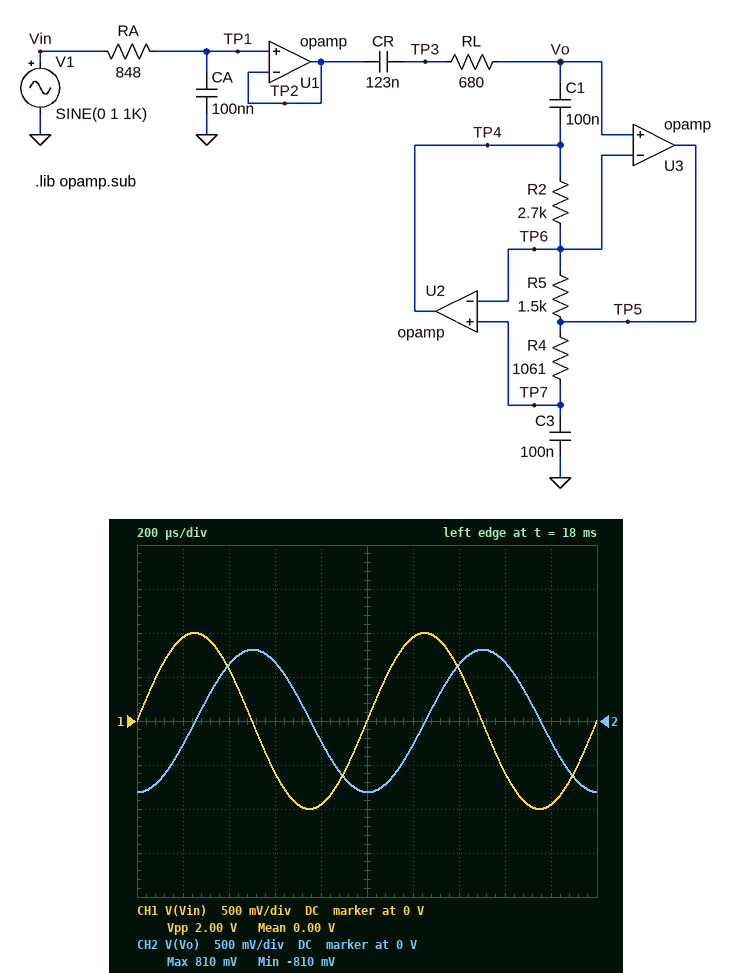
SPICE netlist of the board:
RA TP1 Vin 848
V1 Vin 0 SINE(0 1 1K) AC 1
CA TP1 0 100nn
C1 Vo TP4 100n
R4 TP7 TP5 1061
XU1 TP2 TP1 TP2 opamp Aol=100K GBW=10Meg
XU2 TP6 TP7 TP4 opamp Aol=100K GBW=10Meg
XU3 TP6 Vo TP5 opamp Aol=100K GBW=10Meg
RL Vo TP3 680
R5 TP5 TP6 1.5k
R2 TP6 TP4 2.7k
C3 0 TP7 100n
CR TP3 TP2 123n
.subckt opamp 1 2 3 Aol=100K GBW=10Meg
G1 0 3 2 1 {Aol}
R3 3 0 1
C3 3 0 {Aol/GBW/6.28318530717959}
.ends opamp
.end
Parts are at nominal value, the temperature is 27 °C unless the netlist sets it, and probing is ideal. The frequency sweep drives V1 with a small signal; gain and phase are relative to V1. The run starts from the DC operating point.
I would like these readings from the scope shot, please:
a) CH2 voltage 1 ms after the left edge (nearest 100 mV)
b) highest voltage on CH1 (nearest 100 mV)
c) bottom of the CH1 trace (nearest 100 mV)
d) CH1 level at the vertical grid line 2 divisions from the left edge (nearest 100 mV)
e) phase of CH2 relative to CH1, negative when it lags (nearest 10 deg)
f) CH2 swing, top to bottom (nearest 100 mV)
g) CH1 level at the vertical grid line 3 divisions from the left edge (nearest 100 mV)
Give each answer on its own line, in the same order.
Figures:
-800 mV
1.0 V
-1.0 V
600 mV
-90 deg
1.6 V
-600 mV
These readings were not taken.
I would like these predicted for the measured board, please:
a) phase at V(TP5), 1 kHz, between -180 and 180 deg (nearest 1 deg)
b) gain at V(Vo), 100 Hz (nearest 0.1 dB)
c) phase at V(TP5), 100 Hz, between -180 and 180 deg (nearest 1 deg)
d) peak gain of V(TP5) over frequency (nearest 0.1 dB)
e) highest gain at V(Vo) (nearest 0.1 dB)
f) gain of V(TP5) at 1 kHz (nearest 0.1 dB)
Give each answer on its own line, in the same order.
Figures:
-58 deg
0 dB
-5 deg
0.2 dB
0 dB
-0.2 dB
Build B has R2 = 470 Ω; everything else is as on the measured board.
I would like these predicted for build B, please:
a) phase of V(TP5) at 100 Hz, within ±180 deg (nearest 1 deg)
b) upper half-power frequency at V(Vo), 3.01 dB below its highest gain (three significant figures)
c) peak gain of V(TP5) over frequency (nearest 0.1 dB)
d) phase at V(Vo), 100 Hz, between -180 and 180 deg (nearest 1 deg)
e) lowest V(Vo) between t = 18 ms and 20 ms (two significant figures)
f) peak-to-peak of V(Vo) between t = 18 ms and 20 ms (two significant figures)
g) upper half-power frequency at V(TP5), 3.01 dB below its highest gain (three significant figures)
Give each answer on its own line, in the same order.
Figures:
0 deg
3.65 kHz
6.8 dB
-4 deg
-950 mV
1.9 V
3.96 kHz
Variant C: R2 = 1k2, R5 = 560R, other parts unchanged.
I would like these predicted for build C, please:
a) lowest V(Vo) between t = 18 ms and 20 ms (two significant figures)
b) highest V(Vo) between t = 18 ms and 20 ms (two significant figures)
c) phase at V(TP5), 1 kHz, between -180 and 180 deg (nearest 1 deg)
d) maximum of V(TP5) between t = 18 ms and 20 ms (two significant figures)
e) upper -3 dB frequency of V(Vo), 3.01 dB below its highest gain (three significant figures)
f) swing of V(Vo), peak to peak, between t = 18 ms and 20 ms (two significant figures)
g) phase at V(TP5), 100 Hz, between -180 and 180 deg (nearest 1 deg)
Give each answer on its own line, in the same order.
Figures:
-720 mV
720 mV
-66 deg
870 mV
1.02 kHz
1.4 V
-6 deg
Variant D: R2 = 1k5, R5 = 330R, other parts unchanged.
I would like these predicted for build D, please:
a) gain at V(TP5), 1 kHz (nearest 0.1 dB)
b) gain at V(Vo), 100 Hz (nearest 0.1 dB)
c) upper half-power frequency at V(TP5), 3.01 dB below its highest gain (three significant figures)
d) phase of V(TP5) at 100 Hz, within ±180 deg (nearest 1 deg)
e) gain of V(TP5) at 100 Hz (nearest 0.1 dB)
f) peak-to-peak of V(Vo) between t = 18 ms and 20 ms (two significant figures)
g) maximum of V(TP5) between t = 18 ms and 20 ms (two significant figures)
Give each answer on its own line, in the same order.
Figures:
-7.4 dB
-0.2 dB
524 Hz
-13 deg
-0.1 dB
710 mV
430 mV
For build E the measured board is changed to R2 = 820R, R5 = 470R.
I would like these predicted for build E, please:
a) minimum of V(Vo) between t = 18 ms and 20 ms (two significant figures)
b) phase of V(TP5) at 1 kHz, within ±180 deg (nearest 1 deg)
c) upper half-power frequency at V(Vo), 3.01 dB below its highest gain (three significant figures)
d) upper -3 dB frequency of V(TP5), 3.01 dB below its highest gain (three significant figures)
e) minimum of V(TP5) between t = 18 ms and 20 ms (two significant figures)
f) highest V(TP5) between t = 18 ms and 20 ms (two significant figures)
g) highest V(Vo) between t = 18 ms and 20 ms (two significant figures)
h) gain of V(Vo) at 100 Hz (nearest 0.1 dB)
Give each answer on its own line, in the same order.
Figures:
-820 mV
-56 deg
1.22 kHz
1.59 kHz
-990 mV
990 mV
820 mV
0 dB
